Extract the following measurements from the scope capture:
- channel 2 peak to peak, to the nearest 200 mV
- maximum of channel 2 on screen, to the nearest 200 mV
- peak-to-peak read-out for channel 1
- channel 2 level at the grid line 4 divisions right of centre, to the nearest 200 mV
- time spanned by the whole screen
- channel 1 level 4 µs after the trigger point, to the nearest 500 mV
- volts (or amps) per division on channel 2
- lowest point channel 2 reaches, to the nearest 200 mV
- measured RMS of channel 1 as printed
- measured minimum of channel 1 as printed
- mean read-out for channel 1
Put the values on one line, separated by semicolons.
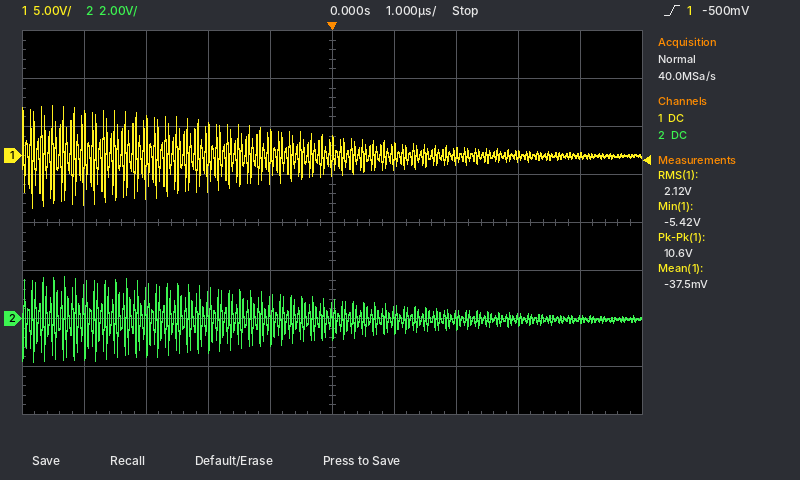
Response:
3.6 V; 1.8 V; 10.6 V; 0.0 V; 10 µs; 0.0 V; 2 V; -1.8 V; 2.12 V; -5.42 V; -37.5 mV
